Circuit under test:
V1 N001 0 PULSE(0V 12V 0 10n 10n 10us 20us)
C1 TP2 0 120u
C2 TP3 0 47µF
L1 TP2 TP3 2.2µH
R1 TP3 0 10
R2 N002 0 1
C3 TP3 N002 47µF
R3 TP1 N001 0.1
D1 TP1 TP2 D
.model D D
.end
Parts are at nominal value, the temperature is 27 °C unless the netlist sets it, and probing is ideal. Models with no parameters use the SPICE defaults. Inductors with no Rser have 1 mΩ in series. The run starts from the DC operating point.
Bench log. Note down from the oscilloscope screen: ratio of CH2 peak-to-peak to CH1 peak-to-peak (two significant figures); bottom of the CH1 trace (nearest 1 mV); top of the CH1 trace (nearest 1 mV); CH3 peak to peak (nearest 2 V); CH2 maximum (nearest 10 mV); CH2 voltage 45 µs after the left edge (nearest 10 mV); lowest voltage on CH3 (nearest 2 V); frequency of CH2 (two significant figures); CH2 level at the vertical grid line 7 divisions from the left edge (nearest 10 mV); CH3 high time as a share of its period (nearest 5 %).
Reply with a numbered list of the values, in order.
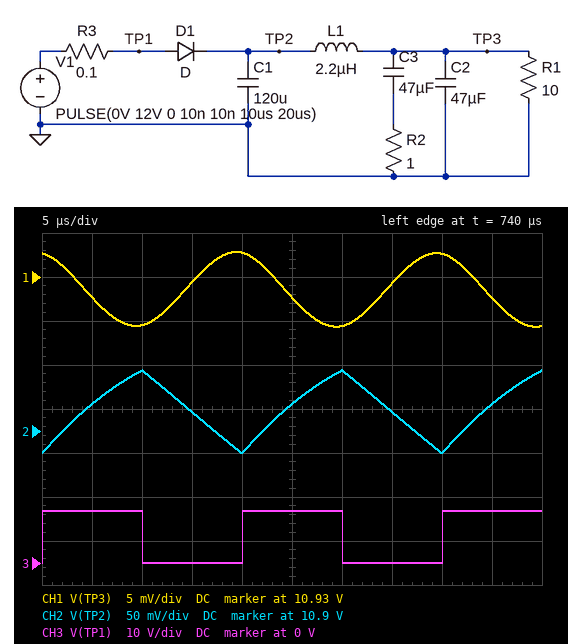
1. 11
2. 10.919 V
3. 10.928 V
4. 12 V
5. 10.97 V
6. 10.93 V
7. 0 V
8. 50 kHz
9. 10.92 V
10. 50 %
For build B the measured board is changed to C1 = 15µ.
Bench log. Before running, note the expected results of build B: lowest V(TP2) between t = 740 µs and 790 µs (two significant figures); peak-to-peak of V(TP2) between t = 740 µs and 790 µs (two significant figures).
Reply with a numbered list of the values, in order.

1. 10 V
2. 980 mV
